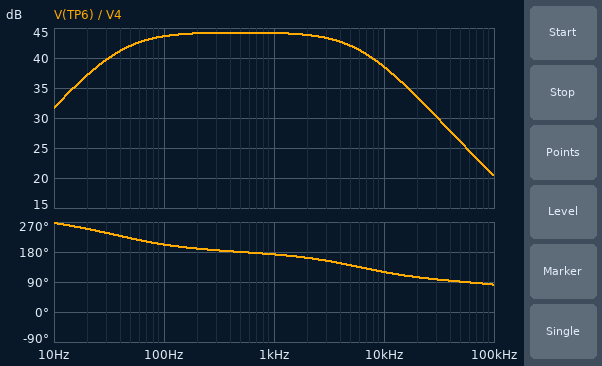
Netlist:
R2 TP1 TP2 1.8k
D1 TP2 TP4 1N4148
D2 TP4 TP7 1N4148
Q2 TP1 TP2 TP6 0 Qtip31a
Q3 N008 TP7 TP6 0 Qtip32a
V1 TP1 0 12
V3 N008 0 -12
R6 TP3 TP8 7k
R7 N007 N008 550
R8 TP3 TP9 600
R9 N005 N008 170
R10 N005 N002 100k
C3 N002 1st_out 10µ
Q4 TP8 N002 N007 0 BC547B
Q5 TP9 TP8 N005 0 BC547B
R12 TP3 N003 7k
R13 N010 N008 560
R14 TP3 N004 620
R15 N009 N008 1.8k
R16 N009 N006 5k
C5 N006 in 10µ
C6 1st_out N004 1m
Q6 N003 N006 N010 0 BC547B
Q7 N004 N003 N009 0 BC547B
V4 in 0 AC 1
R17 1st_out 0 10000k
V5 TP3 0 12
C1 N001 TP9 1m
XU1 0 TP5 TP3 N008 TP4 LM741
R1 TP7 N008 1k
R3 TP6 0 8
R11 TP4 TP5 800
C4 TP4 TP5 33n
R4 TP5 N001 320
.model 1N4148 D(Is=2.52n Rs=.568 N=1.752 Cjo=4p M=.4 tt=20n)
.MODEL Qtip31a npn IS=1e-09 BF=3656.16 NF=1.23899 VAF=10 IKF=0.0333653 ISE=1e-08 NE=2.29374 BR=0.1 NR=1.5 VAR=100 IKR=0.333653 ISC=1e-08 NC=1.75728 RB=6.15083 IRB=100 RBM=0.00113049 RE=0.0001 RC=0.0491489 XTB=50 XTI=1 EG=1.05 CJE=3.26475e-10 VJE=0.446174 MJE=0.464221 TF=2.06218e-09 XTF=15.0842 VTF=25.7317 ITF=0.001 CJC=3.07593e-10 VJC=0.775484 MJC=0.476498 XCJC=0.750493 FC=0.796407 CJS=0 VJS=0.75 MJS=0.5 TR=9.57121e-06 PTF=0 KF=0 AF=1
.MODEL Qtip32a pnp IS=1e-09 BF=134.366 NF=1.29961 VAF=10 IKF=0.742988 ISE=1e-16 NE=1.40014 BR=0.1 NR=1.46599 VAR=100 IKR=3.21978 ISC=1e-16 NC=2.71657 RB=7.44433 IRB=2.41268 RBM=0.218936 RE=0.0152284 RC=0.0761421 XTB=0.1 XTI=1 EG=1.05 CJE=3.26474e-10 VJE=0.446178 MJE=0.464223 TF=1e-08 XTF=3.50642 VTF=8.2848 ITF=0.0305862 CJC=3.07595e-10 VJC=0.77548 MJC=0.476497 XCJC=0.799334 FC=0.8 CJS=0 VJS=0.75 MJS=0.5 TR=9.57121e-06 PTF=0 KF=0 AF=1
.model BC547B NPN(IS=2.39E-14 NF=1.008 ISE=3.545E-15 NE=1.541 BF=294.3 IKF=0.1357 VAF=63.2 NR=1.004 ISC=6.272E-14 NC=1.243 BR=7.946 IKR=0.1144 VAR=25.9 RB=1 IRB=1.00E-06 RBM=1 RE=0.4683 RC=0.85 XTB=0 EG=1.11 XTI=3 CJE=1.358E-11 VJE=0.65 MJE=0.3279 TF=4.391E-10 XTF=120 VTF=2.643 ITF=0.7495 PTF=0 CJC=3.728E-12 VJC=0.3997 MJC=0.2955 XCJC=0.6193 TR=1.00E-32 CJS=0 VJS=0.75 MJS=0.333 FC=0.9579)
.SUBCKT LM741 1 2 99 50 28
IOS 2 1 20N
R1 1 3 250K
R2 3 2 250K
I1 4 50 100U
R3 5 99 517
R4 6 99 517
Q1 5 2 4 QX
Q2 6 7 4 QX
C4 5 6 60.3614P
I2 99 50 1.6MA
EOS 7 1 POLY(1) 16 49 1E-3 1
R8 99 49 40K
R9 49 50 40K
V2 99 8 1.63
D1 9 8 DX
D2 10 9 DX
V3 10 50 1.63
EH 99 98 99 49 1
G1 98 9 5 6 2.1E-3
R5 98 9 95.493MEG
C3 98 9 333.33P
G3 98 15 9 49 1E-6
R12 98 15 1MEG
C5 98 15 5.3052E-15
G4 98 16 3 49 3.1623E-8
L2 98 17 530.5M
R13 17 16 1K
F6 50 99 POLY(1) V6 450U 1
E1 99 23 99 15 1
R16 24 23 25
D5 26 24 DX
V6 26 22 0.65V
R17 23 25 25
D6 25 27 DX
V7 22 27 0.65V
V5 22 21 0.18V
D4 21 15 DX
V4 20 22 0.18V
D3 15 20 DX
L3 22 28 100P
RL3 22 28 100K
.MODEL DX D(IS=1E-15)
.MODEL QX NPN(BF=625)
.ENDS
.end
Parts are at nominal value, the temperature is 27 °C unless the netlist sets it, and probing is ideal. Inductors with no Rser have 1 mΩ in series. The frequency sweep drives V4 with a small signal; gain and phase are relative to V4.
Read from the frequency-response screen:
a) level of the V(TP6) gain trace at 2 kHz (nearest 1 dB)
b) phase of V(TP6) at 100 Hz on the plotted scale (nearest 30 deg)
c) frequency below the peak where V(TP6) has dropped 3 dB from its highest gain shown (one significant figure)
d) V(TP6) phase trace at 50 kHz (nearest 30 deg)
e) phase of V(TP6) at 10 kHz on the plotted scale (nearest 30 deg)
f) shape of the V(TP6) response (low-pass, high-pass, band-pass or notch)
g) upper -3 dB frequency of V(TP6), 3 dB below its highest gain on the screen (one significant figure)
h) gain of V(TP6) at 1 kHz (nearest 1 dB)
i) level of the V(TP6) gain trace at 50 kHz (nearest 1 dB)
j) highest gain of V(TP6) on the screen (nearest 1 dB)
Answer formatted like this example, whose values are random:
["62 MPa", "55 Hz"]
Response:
["44 dB", "210 deg", "40 Hz", "90 deg", "120 deg", "band-pass", "6 kHz", "44 dB", "26 dB", "44 dB"]
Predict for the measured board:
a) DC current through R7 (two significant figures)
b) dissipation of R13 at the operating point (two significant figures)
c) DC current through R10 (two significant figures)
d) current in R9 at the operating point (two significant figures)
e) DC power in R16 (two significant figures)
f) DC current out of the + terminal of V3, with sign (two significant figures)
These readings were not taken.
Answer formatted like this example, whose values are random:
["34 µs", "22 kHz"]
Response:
["2.8 mA", "5.0 mW", "9.8 µA", "19 mA", "560 nW", "-460 mA"]
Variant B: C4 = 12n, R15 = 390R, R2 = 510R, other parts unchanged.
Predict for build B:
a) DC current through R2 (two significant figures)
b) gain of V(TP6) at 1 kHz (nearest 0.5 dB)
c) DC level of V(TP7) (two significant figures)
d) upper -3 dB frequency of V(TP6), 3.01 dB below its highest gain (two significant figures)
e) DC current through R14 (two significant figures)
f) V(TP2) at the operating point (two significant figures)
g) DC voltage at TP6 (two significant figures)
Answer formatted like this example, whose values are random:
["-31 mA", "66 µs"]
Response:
["22 mA", "55.0 dB", "-680 mV", "16 kHz", "6.1 mA", "730 mV", "18 mV"]
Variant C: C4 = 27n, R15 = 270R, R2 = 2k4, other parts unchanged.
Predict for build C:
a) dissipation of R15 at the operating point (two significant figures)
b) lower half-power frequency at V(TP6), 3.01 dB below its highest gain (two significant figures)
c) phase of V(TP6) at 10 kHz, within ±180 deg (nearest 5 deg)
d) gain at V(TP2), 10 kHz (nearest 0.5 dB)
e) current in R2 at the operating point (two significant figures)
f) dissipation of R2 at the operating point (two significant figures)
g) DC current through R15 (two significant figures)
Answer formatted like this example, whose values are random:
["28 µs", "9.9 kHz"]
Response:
["21 mW", "38 Hz", "125 deg", "53.5 dB", "4.7 mA", "54 mW", "8.8 mA"]
